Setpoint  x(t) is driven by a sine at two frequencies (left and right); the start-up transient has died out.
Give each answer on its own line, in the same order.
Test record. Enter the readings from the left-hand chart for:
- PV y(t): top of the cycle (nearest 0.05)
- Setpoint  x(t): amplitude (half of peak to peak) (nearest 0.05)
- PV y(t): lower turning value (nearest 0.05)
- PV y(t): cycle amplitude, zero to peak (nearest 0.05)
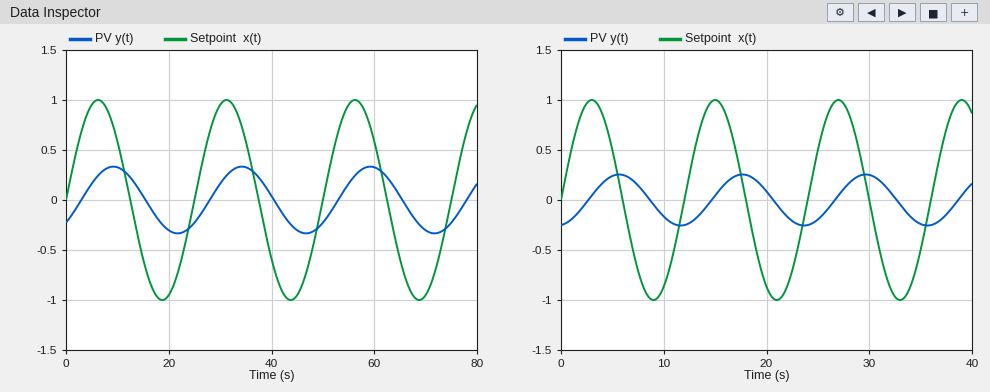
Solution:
0.35
1.00
-0.35
0.35
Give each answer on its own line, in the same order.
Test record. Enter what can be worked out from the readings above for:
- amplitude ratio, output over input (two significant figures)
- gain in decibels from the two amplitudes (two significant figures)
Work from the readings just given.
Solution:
0.35
-9.1 dB
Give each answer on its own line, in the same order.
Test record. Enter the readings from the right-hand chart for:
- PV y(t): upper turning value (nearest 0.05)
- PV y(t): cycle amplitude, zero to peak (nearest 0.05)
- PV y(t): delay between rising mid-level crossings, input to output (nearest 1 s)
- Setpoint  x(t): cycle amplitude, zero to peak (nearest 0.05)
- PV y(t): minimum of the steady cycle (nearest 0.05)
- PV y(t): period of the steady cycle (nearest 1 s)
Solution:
0.25
0.25
3 s
1.00
-0.25
12 s
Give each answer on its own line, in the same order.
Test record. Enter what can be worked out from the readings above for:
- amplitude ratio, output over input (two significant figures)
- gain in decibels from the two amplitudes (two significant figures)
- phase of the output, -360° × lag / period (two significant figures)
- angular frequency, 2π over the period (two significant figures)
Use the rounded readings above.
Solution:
0.25
-12 dB
-90°
0.52 rad/s
